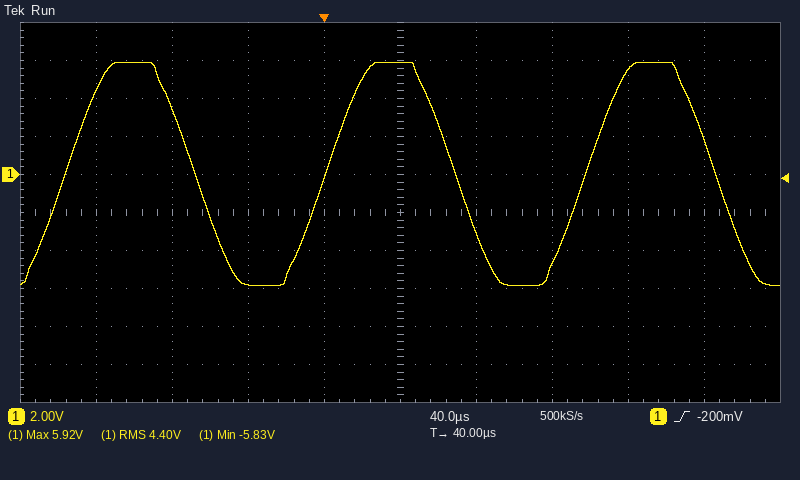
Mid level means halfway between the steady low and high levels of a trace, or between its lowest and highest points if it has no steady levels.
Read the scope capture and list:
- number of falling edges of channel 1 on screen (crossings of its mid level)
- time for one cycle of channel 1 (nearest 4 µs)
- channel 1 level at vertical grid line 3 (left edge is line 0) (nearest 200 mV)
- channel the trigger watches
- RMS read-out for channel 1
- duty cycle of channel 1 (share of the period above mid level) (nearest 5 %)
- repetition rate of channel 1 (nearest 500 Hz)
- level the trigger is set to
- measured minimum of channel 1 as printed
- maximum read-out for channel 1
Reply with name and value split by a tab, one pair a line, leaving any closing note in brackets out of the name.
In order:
number of falling edges of channel 1 on screen	3
time for one cycle of channel 1	136 µs
channel 1 level at vertical grid line 3 (left edge is line 0)	-5.8 V
channel the trigger watches	channel 1
RMS read-out for channel 1	4.40 V
duty cycle of channel 1 (share of the period above mid level)	50 %
repetition rate of channel 1	7.5 kHz
level the trigger is set to	-200 mV
measured minimum of channel 1 as printed	-5.83 V
maximum read-out for channel 1	5.92 V
